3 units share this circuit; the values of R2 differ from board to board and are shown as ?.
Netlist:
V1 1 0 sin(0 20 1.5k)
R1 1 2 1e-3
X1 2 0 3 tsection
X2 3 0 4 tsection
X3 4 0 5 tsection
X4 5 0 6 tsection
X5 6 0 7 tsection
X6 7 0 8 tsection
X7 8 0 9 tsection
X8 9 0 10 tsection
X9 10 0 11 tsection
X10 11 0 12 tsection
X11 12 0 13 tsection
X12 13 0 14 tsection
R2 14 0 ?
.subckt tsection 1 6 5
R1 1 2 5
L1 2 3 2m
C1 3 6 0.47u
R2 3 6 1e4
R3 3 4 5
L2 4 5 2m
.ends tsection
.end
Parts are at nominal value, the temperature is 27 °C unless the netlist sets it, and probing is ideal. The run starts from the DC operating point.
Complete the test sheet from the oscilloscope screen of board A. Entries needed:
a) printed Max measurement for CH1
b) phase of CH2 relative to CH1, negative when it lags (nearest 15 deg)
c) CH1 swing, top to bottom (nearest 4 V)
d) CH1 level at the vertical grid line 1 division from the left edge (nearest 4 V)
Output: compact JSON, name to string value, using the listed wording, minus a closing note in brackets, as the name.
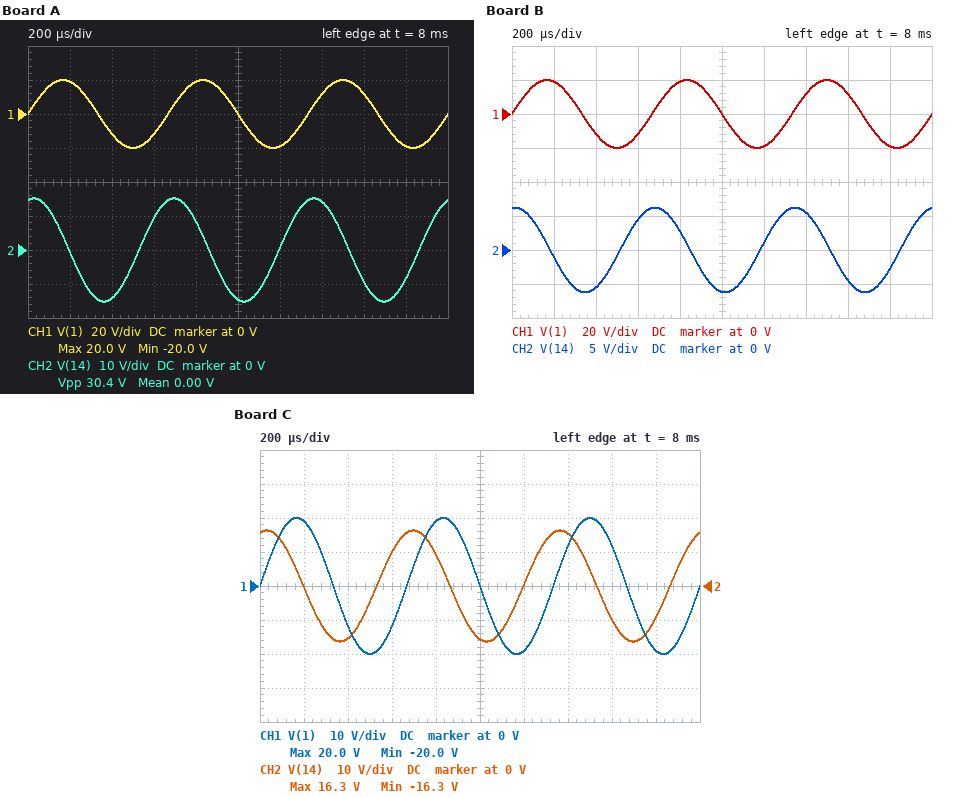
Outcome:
{"printed Max measurement for CH1": "20.0 V", "phase of CH2 relative to CH1, negative when it lags": "75 deg", "CH1 swing, top to bottom": "40 V", "CH1 level at the vertical grid line 1 division from the left edge": "20 V"}
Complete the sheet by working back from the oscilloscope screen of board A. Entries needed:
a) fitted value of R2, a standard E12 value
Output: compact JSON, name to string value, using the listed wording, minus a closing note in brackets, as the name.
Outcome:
{"fitted value of R2, a standard E12 value": "220 Ω"}
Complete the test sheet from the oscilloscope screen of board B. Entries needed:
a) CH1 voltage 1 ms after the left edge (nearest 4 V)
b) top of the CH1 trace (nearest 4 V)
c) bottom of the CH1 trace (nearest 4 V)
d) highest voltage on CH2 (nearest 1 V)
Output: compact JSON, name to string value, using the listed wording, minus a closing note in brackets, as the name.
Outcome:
{"CH1 voltage 1 ms after the left edge": "0 V", "top of the CH1 trace": "20 V", "bottom of the CH1 trace": "-20 V", "highest voltage on CH2": "6 V"}
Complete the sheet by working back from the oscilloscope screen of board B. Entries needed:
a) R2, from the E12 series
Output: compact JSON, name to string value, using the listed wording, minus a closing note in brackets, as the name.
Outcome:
{"R2, from the E12 series": "47 Ω"}
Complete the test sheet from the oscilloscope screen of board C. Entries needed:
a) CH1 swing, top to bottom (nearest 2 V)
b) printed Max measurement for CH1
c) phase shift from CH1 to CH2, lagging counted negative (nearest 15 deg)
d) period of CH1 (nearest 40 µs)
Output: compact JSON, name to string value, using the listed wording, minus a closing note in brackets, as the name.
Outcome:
{"CH1 swing, top to bottom": "40 V", "printed Max measurement for CH1": "20.0 V", "phase shift from CH1 to CH2, lagging counted negative": "75 deg", "period of CH1": "680 µs"}
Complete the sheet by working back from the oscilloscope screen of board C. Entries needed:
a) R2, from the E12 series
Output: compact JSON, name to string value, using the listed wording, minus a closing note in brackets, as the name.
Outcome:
{"R2, from the E12 series": "270 Ω"}
